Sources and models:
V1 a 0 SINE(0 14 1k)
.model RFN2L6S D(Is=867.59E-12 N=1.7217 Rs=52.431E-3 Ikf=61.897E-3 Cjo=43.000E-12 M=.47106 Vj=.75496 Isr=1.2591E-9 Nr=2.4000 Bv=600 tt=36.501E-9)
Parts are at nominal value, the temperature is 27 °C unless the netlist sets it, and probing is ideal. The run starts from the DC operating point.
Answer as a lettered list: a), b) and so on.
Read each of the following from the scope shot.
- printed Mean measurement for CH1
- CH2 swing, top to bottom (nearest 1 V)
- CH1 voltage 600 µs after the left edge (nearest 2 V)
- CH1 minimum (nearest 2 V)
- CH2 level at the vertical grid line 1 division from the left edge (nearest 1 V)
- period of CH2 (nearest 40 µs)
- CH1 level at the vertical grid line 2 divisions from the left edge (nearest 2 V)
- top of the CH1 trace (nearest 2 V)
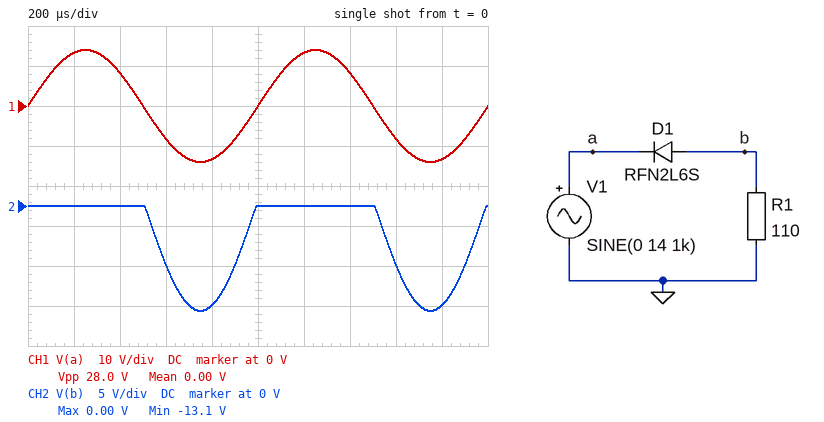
a) 0.00 V
b) 13 V
c) -8 V
d) -14 V
e) 0 V
f) 1.00 ms
g) 8 V
h) 14 V
